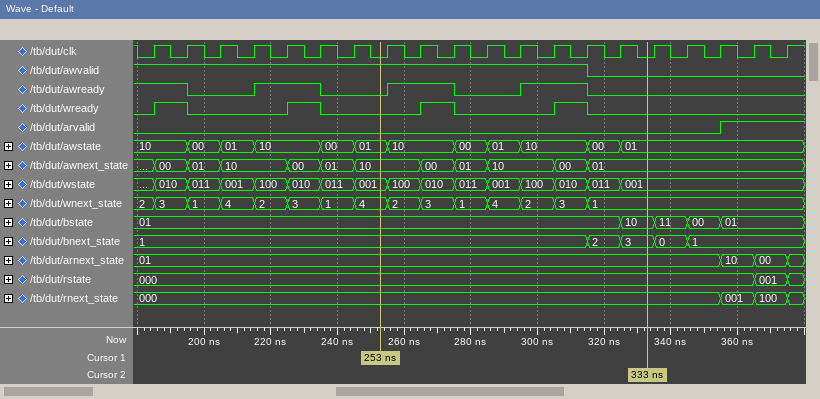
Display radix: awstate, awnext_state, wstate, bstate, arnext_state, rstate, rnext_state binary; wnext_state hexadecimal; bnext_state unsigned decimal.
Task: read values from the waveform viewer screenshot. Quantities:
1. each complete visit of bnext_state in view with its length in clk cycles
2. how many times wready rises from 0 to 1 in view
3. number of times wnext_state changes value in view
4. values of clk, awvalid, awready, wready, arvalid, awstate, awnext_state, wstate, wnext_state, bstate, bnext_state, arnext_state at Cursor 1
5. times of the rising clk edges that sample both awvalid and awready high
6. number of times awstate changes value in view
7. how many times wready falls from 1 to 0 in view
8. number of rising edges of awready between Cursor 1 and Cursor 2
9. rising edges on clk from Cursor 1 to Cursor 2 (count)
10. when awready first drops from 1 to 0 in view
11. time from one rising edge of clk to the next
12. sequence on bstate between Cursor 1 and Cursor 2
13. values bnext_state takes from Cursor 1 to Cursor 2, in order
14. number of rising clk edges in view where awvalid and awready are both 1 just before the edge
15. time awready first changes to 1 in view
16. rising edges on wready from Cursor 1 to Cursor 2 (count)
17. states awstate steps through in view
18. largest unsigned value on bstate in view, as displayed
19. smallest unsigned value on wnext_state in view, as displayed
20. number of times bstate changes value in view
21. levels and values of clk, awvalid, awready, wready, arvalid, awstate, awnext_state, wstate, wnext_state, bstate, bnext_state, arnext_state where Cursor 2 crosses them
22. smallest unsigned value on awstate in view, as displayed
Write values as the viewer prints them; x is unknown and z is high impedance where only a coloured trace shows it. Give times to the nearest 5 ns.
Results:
2: 1, 3: 1, 0: 1
4
14
clk=0, awvalid=1, awready=0, wready=0, arvalid=0, awstate=01, awnext_state=10, wstate=001, wnext_state=4, bstate=01, bnext_state=1, arnext_state=01
185 ns, 195 ns, 225 ns, 235 ns, 265 ns, 275 ns, 305 ns, 315 ns
11
4
2
8
195 ns
10 ns
01, 10
1, 2, 3
8
215 ns
2
10, 00, 01, 10, 00, 01, 10, 00, 01, 10, 00, 01
11
1
4
clk=0, awvalid=0, awready=0, wready=0, arvalid=0, awstate=01, awnext_state=01, wstate=001, wnext_state=1, bstate=10, bnext_state=3, arnext_state=01
00
